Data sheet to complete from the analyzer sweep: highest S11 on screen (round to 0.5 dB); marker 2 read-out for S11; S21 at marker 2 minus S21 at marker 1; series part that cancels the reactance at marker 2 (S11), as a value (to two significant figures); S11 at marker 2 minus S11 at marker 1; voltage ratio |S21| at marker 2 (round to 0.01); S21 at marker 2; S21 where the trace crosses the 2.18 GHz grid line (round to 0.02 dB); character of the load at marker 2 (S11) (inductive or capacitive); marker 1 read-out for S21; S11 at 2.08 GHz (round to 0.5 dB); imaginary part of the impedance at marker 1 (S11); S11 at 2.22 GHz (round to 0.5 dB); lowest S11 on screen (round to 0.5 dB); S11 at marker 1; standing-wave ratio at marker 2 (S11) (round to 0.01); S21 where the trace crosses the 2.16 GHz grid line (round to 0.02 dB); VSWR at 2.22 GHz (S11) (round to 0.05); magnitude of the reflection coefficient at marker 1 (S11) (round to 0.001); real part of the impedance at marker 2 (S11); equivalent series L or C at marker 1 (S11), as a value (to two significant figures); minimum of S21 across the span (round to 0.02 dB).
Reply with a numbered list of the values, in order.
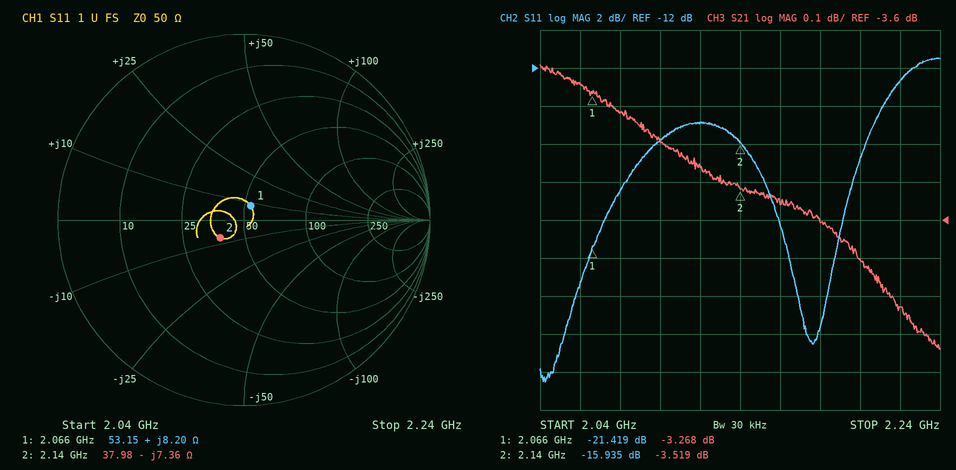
1. -11.5 dB
2. -15.935 dB
3. -0.251 dB
4. 550 pH
5. 5.484 dB
6. 0.67
7. -3.519 dB
8. -3.60 dB
9. capacitive
10. -3.268 dB
11. -18.5 dB
12. +8.20 Ω
13. -12.5 dB
14. -28.5 dB
15. -21.419 dB
16. 1.38
17. -3.56 dB
18. 1.60
19. 0.085
20. 37.98 Ω
21. 630 pH
22. -3.94 dB
